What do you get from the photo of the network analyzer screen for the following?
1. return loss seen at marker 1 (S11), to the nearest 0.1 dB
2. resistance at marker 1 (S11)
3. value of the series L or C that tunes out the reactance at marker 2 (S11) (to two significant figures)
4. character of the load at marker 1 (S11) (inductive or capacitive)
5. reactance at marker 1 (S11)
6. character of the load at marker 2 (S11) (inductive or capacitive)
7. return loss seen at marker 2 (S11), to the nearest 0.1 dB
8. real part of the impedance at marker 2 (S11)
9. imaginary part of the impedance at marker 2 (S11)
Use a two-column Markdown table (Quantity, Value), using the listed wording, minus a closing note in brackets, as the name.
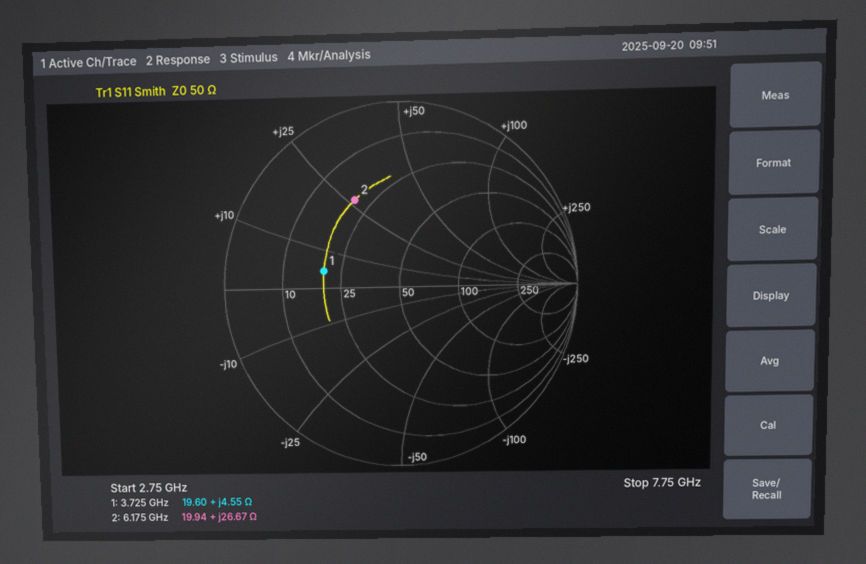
| Quantity | Value |
|---|---|
| return loss seen at marker 1 (S11), to the nearest 0.1 dB | 7.1 dB |
| resistance at marker 1 | 19.60 Ω |
| value of the series L or C that tunes out the reactance at marker 2 (S11) | 970 fF |
| character of the load at marker 1 (S11) | inductive |
| reactance at marker 1 | +4.55 Ω |
| character of the load at marker 2 (S11) | inductive |
| return loss seen at marker 2 (S11), to the nearest 0.1 dB | 5.4 dB |
| real part of the impedance at marker 2 | 19.94 Ω |
| imaginary part of the impedance at marker 2 | +26.67 Ω |
